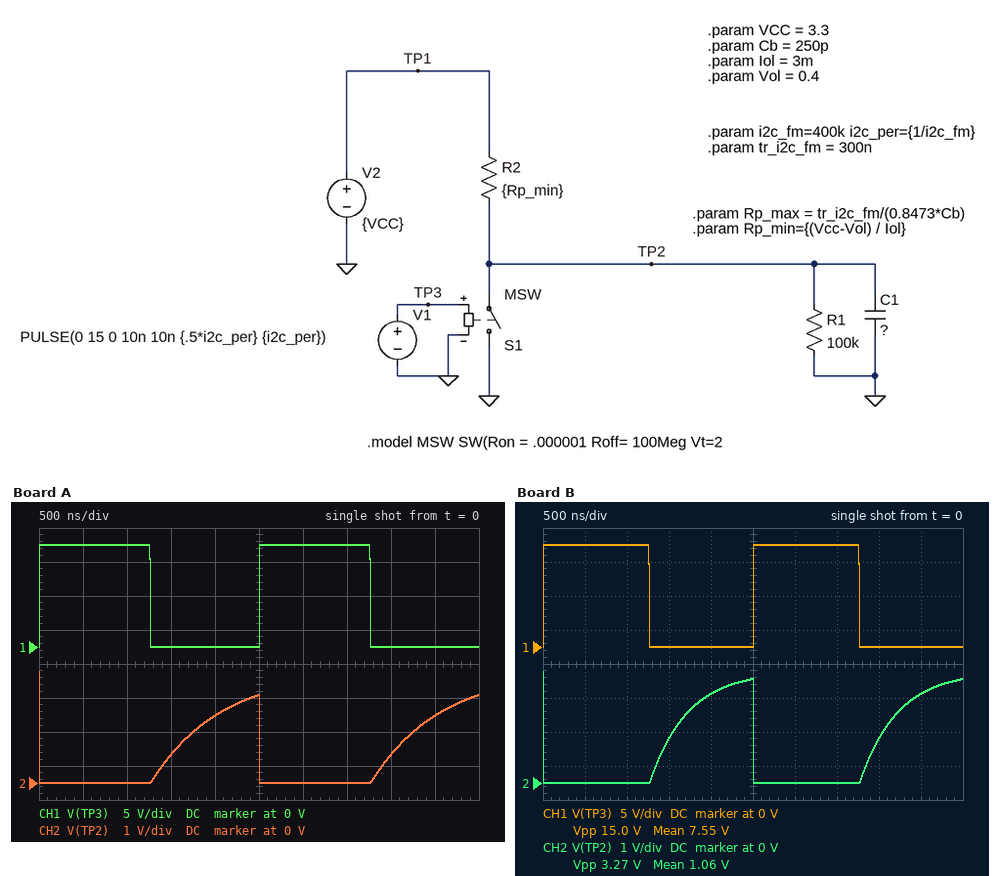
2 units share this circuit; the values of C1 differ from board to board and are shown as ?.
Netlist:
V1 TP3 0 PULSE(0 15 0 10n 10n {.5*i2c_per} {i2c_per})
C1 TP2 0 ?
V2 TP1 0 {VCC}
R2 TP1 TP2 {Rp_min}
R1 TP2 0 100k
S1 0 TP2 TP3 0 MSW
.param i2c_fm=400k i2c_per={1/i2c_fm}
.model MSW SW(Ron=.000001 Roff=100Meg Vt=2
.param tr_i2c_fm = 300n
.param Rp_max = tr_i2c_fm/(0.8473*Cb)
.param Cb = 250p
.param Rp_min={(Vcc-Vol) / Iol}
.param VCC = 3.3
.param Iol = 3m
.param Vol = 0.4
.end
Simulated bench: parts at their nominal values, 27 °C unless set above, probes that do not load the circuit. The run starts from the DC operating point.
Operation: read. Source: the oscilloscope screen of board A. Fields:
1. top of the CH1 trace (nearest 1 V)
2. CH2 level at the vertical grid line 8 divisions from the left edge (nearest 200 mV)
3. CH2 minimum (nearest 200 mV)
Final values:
15 V
800 mV
0 V
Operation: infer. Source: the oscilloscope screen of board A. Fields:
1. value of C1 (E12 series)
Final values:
820 pF
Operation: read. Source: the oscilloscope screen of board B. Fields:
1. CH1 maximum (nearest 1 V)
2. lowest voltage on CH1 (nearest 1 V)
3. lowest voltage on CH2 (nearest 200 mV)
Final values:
15 V
0 V
0 V
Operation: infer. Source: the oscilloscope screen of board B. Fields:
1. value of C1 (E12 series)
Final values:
470 pF
